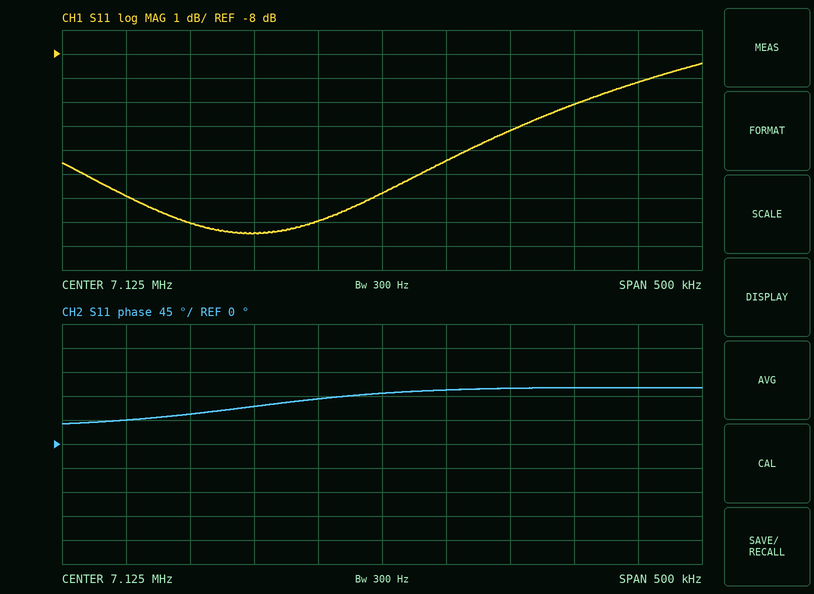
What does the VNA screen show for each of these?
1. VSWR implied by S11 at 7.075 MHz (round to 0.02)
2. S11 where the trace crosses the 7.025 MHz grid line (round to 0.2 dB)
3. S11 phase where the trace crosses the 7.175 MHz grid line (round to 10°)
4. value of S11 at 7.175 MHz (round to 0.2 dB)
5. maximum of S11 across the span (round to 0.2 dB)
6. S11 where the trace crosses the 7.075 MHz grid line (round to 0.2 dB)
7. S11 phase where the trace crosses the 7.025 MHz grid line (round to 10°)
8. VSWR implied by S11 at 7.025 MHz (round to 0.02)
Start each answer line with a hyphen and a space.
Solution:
- 1.44
- -15.4 dB
- 100°
- -12.4 dB
- -8.4 dB
- -15.0 dB
- 70°
- 1.40
